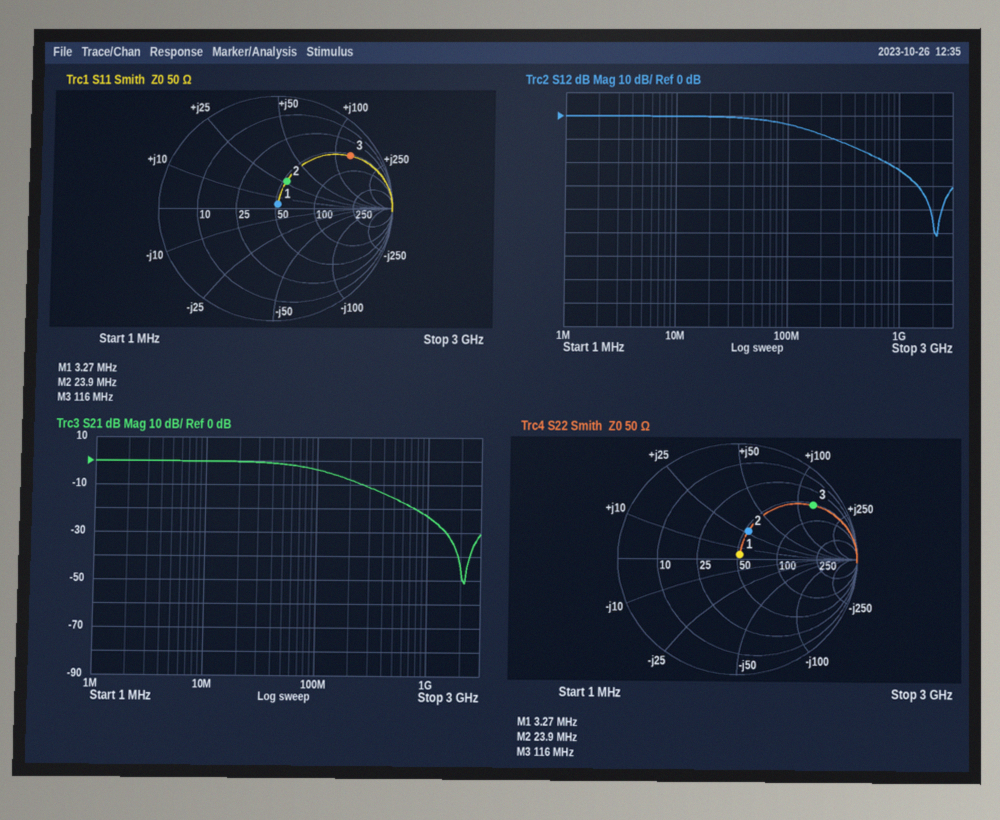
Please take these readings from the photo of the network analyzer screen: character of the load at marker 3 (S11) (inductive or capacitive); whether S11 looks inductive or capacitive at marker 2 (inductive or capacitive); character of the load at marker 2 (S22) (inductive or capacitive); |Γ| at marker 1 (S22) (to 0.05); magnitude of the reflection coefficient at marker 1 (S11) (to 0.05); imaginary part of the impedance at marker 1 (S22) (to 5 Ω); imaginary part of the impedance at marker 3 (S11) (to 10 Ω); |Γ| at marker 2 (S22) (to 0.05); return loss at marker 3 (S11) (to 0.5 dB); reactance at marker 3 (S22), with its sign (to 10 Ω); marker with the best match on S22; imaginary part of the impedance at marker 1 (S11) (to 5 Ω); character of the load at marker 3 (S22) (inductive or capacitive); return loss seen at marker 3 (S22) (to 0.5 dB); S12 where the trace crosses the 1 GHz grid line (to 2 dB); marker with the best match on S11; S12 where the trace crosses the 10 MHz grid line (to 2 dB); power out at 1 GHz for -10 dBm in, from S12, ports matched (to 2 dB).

inductive
inductive
inductive
0.05
0.05
+5 Ω
+130 Ω
0.25
2.0 dB
+130 Ω
marker 1
+5 Ω
inductive
2.0 dB
-24 dB
marker 1
0 dB
-34 dBm
